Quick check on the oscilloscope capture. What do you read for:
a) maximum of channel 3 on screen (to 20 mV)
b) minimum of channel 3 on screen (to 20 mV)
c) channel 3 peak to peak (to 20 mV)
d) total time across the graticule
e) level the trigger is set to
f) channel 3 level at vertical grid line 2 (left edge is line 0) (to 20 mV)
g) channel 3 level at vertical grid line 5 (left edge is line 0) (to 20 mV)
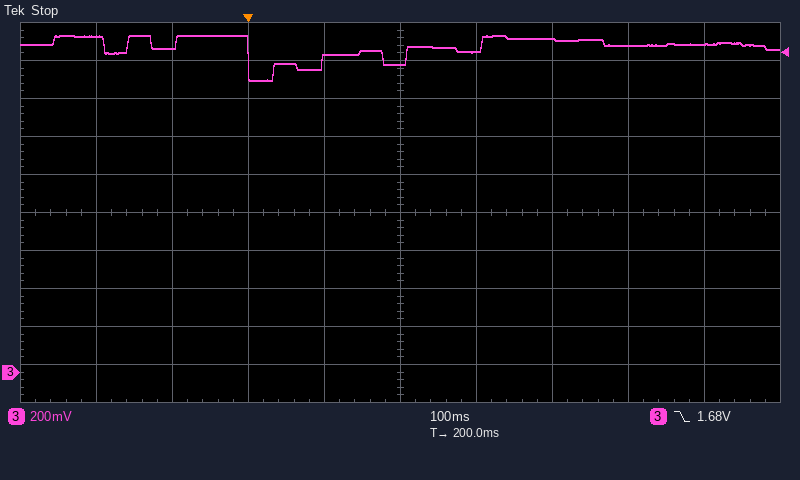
1.78 V
1.54 V
240 mV
1 s
1.68 V
1.72 V
1.62 V
